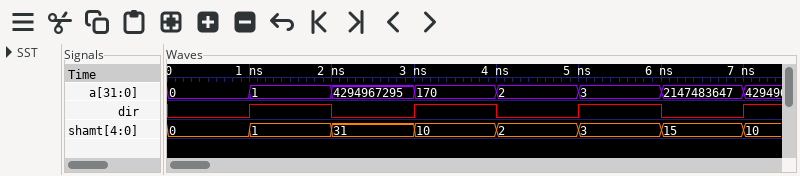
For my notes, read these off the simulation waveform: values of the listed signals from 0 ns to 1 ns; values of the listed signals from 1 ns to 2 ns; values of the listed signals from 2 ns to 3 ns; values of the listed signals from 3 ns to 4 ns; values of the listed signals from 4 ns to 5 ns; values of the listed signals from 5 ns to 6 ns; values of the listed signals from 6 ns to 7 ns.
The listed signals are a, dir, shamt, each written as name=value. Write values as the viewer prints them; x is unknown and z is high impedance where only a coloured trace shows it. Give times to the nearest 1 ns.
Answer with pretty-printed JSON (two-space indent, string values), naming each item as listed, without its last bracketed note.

{
  "values of the listed signals from 0 ns to 1 ns": "a=0, dir=0, shamt=0",
  "values of the listed signals from 1 ns to 2 ns": "a=1, dir=1, shamt=1",
  "values of the listed signals from 2 ns to 3 ns": "a=4294967295, dir=0, shamt=31",
  "values of the listed signals from 3 ns to 4 ns": "a=170, dir=1, shamt=10",
  "values of the listed signals from 4 ns to 5 ns": "a=2, dir=0, shamt=2",
  "values of the listed signals from 5 ns to 6 ns": "a=3, dir=1, shamt=3",
  "values of the listed signals from 6 ns to 7 ns": "a=2147483647, dir=0, shamt=15"
}
